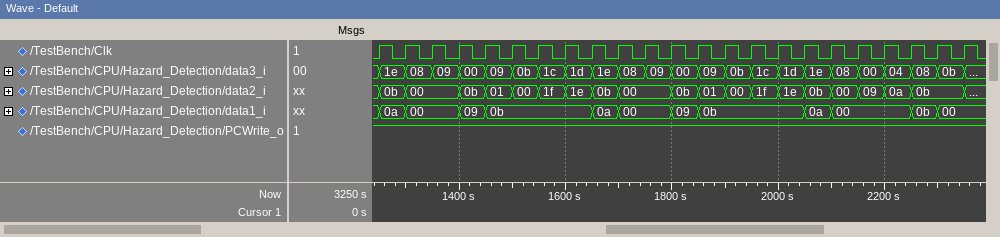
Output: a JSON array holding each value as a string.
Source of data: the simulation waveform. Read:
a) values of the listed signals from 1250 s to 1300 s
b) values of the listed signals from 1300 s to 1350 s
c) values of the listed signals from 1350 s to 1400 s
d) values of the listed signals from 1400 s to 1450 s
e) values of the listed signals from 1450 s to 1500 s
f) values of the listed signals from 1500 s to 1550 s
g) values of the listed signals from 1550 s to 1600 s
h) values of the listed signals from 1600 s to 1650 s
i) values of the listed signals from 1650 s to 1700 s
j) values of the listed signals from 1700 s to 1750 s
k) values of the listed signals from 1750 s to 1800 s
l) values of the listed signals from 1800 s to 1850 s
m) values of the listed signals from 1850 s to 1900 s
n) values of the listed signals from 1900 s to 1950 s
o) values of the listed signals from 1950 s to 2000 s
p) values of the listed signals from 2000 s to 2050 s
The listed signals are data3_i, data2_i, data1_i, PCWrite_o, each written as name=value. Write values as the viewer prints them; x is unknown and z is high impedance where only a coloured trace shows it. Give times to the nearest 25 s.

["data3_i=1e, data2_i=0b, data1_i=0a, PCWrite_o=1", "data3_i=08, data2_i=00, data1_i=00, PCWrite_o=1", "data3_i=09, data2_i=00, data1_i=00, PCWrite_o=1", "data3_i=00, data2_i=0b, data1_i=09, PCWrite_o=1", "data3_i=09, data2_i=01, data1_i=0b, PCWrite_o=1", "data3_i=0b, data2_i=00, data1_i=0b, PCWrite_o=1", "data3_i=1c, data2_i=1f, data1_i=0b, PCWrite_o=1", "data3_i=1d, data2_i=1e, data1_i=0b, PCWrite_o=1", "data3_i=1e, data2_i=0b, data1_i=0a, PCWrite_o=1", "data3_i=08, data2_i=00, data1_i=00, PCWrite_o=1", "data3_i=09, data2_i=00, data1_i=00, PCWrite_o=1", "data3_i=00, data2_i=0b, data1_i=09, PCWrite_o=1", "data3_i=09, data2_i=01, data1_i=0b, PCWrite_o=1", "data3_i=0b, data2_i=00, data1_i=0b, PCWrite_o=1", "data3_i=1c, data2_i=1f, data1_i=0b, PCWrite_o=1", "data3_i=1d, data2_i=1e, data1_i=0b, PCWrite_o=1"]
